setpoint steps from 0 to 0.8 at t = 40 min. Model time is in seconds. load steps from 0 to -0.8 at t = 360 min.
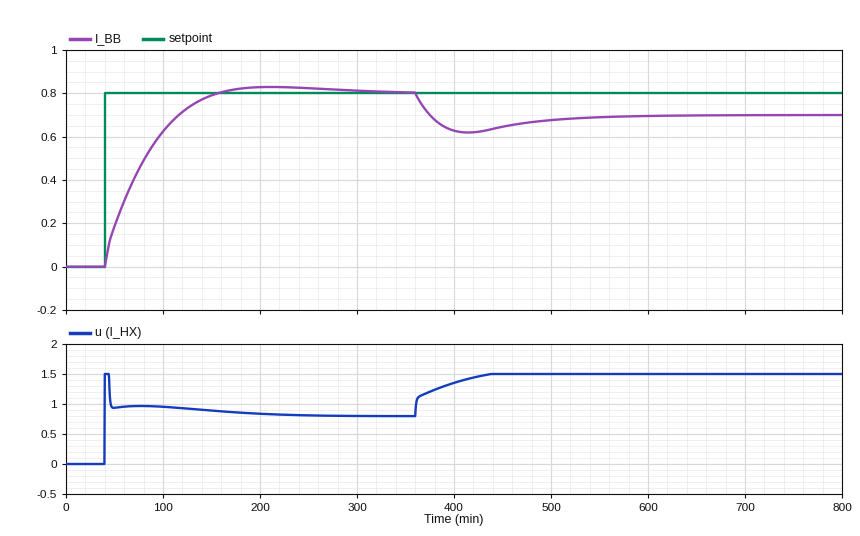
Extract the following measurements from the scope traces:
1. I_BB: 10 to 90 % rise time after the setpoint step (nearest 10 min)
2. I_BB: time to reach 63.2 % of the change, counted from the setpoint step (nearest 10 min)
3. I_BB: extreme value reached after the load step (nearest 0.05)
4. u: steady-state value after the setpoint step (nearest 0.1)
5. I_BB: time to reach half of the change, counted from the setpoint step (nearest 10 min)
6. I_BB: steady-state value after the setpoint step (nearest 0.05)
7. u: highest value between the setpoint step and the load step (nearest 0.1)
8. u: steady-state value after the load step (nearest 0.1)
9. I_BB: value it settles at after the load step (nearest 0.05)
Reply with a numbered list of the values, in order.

1. 80 min
2. 40 min
3. 0.60
4. 0.8
5. 30 min
6. 0.80
7. 1.5
8. 1.5
9. 0.70
